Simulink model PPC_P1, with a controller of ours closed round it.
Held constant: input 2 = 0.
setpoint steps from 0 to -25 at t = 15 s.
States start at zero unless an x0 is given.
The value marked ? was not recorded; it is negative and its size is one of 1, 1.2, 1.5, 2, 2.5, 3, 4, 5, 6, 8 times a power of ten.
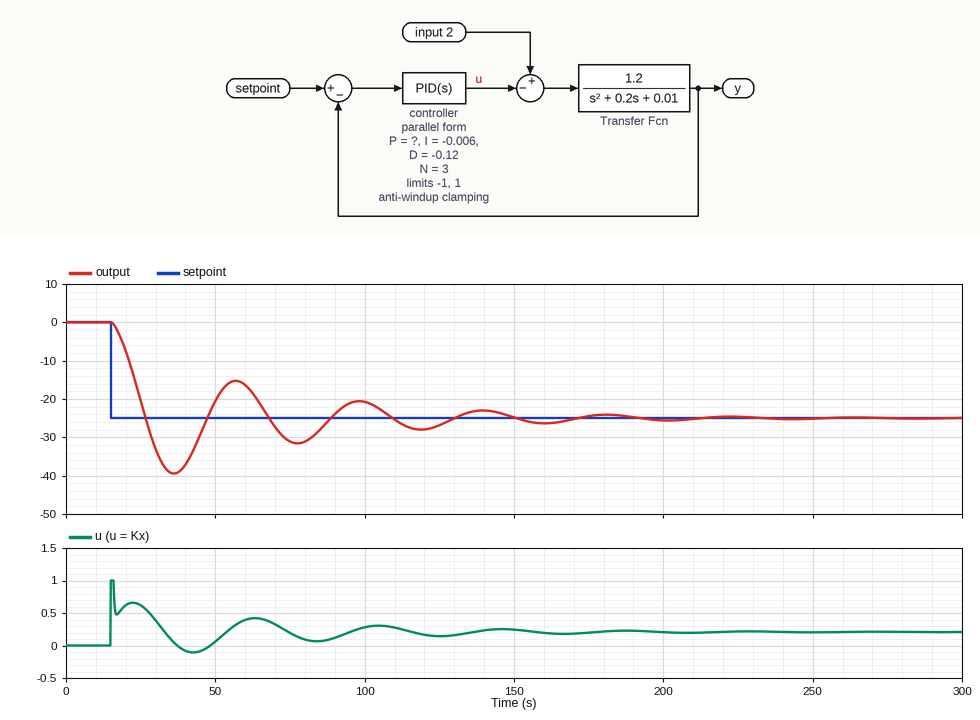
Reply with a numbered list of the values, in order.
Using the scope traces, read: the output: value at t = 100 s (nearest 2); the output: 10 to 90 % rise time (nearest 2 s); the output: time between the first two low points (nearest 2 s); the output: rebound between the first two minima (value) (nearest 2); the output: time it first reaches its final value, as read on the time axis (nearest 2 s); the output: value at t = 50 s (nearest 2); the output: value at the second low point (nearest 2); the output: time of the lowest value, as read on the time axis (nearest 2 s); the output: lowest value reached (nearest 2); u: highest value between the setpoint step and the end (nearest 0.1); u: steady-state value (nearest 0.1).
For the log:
1. -20
2. 8 s
3. 42 s
4. -16
5. 26 s
6. -20
7. -32
8. 36 s
9. -40
10. 1.0
11. 0.2
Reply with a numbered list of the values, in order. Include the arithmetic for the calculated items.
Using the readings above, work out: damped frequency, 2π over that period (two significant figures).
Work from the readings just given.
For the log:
1. 2π / 42 = 0.15 rad/s
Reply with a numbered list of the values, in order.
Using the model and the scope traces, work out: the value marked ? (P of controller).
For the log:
1. -0.02
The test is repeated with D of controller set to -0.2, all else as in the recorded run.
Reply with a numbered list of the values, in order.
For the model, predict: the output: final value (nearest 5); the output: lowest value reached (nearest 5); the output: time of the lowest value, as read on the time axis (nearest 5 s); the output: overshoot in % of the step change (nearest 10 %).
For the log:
1. -25
2. -40
3. 40 s
4. 50 %
